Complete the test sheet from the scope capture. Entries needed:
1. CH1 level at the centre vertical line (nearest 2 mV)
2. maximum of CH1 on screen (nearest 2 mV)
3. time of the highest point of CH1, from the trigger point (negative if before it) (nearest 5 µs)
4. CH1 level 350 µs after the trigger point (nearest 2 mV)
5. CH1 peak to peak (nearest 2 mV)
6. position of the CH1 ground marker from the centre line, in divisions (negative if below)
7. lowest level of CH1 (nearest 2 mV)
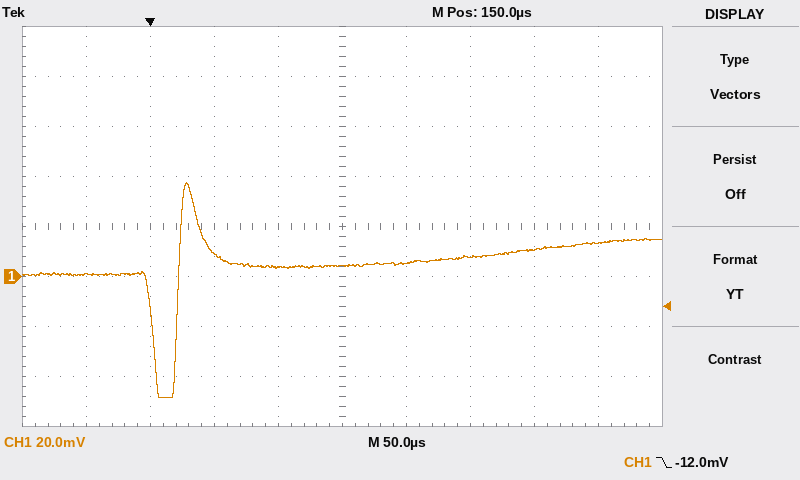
4 mV
38 mV
+30 µs
14 mV
86 mV
-1.0 div
-48 mV
